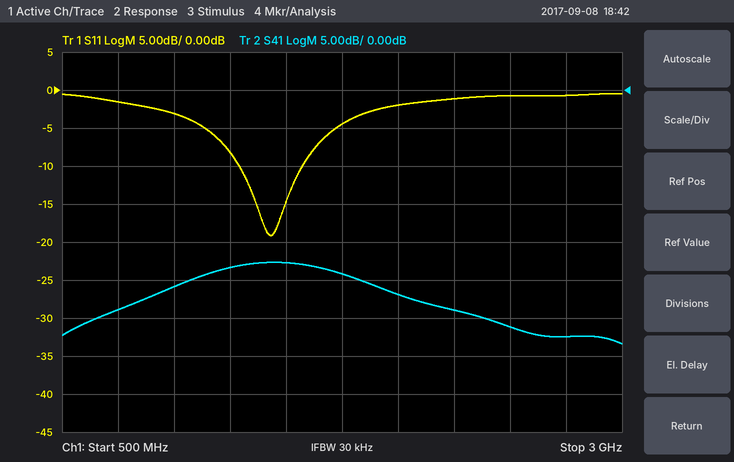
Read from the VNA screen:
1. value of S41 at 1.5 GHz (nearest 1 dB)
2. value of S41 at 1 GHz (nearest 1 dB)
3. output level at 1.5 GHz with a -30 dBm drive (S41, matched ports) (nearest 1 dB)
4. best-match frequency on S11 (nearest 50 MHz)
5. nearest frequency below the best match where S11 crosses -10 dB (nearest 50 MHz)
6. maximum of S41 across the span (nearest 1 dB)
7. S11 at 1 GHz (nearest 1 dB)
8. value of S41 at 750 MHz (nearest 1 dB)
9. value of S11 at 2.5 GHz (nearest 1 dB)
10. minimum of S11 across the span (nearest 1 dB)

-23 dB
-26 dB
-53 dBm
1.45 GHz
1.30 GHz
-23 dB
-3 dB
-29 dB
-1 dB
-19 dB
